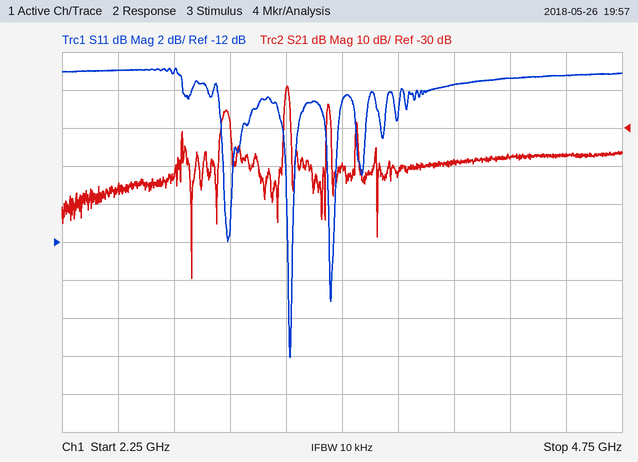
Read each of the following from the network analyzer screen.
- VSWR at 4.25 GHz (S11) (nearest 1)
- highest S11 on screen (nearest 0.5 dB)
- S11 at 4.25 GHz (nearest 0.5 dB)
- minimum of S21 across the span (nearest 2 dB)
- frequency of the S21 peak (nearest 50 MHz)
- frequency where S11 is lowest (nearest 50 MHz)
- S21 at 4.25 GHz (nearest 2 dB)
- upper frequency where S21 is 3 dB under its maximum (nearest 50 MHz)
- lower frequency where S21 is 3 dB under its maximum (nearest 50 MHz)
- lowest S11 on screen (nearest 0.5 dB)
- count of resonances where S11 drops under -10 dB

5
-3.0 dB
-3.5 dB
-70 dB
3.25 GHz
3.25 GHz
-38 dB
3.25 GHz
3.25 GHz
-18.0 dB
3
